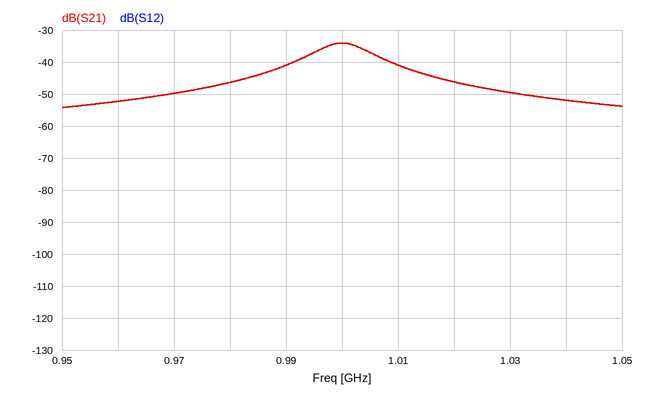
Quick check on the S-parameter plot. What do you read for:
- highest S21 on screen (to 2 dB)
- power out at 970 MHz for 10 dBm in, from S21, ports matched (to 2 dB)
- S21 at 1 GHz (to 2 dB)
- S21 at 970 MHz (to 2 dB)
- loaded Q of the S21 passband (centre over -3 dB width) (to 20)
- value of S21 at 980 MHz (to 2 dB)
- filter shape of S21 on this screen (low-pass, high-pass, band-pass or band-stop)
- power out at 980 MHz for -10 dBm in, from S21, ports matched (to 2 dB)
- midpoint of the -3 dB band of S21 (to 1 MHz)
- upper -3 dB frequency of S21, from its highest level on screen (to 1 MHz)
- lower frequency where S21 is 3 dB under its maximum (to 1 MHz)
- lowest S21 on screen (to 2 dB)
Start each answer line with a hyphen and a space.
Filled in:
- -34 dB
- -40 dBm
- -34 dB
- -50 dB
- 100
- -46 dB
- band-pass
- -56 dBm
- 1.000 GHz
- 1.005 GHz
- 995 MHz
- -54 dB
